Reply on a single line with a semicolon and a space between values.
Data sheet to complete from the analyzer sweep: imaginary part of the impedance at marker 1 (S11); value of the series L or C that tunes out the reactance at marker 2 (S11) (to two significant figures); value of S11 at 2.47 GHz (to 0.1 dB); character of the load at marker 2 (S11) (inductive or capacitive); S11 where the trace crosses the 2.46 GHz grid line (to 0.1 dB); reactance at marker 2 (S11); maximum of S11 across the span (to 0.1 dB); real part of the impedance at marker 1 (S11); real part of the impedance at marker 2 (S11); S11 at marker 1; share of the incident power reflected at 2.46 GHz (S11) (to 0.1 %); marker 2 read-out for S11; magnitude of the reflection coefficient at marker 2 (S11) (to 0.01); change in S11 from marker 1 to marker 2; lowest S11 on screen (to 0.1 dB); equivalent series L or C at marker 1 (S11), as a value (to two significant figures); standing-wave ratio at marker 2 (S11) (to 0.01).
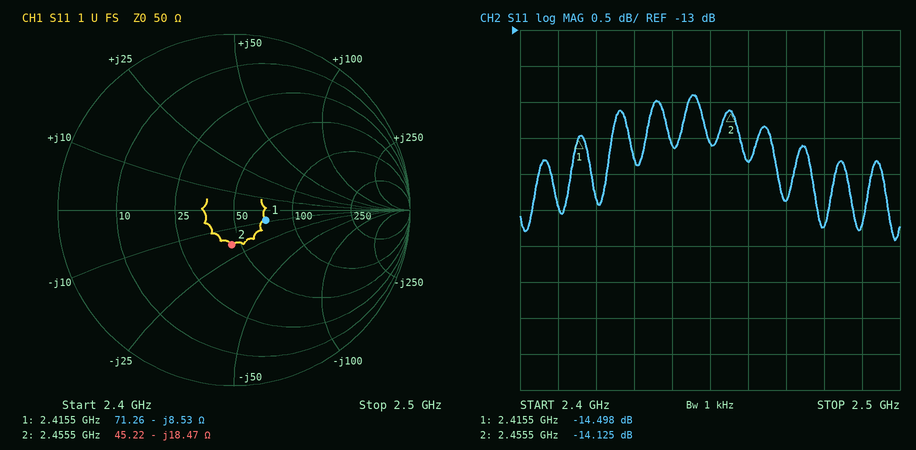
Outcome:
-8.53 Ω; 1.2 nH; -15.4 dB; capacitive; -14.8 dB; -18.47 Ω; -13.9 dB; 71.26 Ω; 45.22 Ω; -14.498 dB; 3.3 %; -14.125 dB; 0.20; 0.373 dB; -15.9 dB; 7.7 pF; 1.49
